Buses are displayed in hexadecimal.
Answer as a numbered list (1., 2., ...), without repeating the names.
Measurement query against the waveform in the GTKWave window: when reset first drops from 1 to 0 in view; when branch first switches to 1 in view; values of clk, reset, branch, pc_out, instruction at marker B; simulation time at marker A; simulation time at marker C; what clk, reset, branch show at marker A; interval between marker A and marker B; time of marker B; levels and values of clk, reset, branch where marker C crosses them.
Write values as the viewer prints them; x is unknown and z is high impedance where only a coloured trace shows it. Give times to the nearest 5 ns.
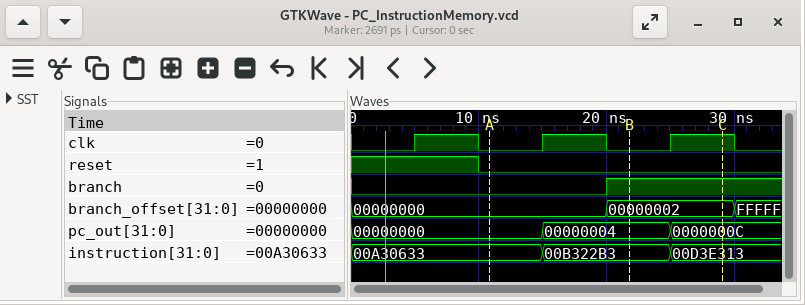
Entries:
1. 10 ns
2. 20 ns
3. clk=0, reset=0, branch=1, pc_out=00000004, instruction=00B322B3
4. 10 ns
5. 30 ns
6. clk=0, reset=0, branch=0
7. 10 ns
8. 20 ns
9. clk=1, reset=0, branch=1
